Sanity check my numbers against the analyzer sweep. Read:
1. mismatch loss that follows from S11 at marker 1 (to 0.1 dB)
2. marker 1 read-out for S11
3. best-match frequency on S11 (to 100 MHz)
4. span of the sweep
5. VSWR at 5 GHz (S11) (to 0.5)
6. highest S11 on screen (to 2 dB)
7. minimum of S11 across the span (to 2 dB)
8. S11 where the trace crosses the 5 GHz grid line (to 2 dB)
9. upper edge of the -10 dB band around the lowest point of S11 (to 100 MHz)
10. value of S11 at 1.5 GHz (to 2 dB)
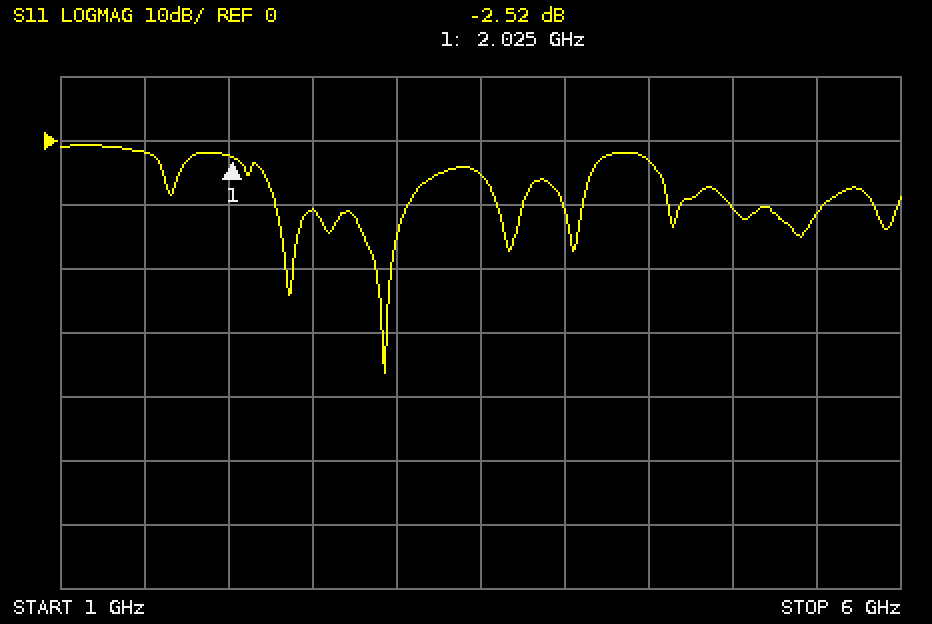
3.6 dB
-2.52 dB
2.9 GHz
5 GHz
2.0
0 dB
-36 dB
-10 dB
3.1 GHz
-2 dB
